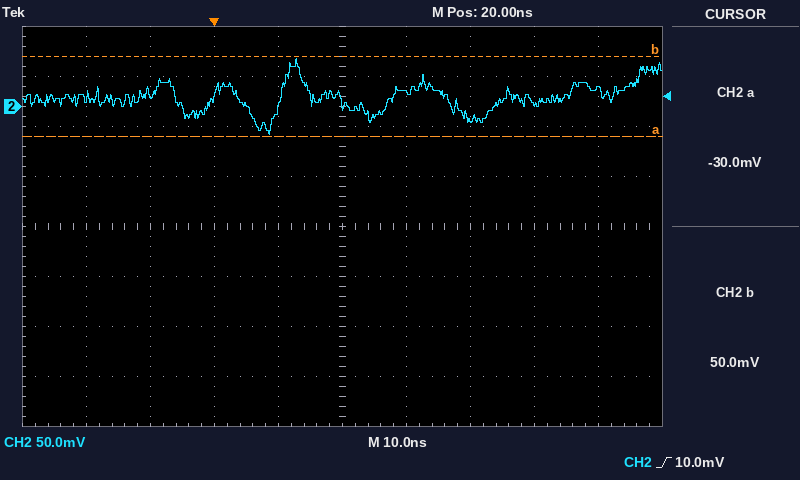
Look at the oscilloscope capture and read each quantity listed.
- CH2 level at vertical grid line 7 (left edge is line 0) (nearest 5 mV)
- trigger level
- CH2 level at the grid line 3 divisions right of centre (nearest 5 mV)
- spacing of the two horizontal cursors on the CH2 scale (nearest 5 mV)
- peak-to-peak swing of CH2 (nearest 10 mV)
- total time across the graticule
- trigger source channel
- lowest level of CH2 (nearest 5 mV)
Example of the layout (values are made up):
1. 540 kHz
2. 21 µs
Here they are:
1. -15 mV
2. 10.0 mV
3. 5 mV
4. 80 mV
5. 80 mV
6. 100 ns
7. CH2
8. -30 mV
